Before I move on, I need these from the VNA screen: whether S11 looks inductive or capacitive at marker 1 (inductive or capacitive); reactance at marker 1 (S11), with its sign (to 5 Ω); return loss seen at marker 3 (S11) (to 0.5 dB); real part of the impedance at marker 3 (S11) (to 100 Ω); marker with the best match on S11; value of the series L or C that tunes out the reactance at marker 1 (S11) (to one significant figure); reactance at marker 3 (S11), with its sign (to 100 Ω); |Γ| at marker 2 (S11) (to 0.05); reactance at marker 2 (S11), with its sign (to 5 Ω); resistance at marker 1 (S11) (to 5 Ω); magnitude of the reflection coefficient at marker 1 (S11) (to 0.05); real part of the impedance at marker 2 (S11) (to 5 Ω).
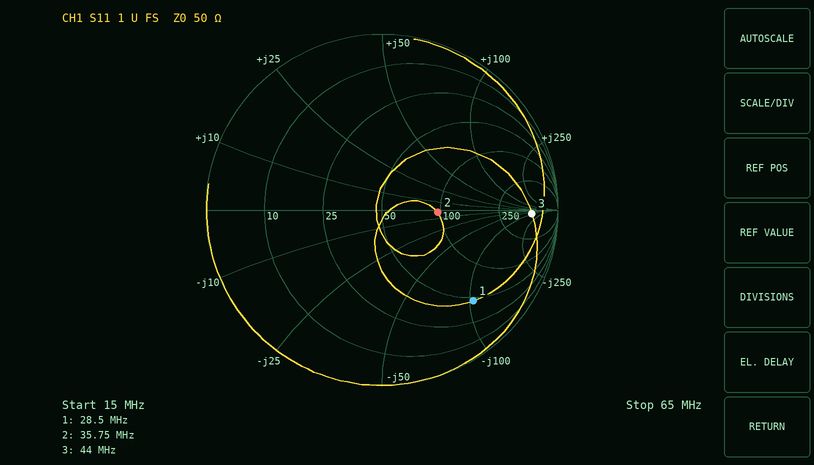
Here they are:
capacitive
-105 Ω
1.5 dB
600 Ω
marker 2
600 nH
-100 Ω
0.30
-5 Ω
45 Ω
0.75
95 Ω
